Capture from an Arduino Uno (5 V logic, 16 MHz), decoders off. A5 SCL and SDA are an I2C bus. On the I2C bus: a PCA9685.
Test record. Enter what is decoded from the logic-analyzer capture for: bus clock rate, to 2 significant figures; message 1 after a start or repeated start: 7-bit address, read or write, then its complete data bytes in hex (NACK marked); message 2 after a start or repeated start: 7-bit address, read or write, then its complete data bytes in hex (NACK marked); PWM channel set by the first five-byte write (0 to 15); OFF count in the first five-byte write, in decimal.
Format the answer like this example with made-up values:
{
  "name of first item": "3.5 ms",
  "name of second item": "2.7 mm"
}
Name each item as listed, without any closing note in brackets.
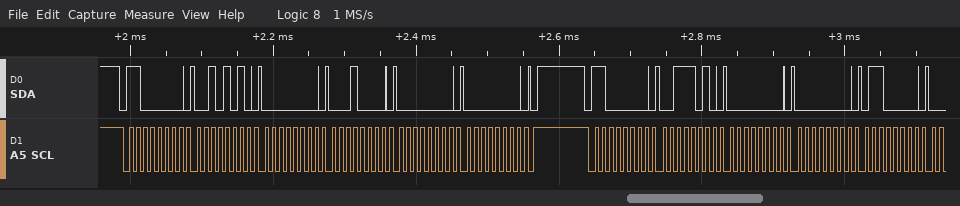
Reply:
{
  "bus clock rate, to 2 significant figures": "100 kHz",
  "message 1 after a start or repeated start: 7-bit address, read or write, then its complete data bytes in hex": "0x60 write: 2A 00 10 00 00",
  "message 2 after a start or repeated start: 7-bit address, read or write, then its complete data bytes in hex": "0x60 write: 3A 00 00 60",
  "PWM channel set by the first five-byte write": "9",
  "OFF count in the first five-byte write, in decimal": "0"
}
